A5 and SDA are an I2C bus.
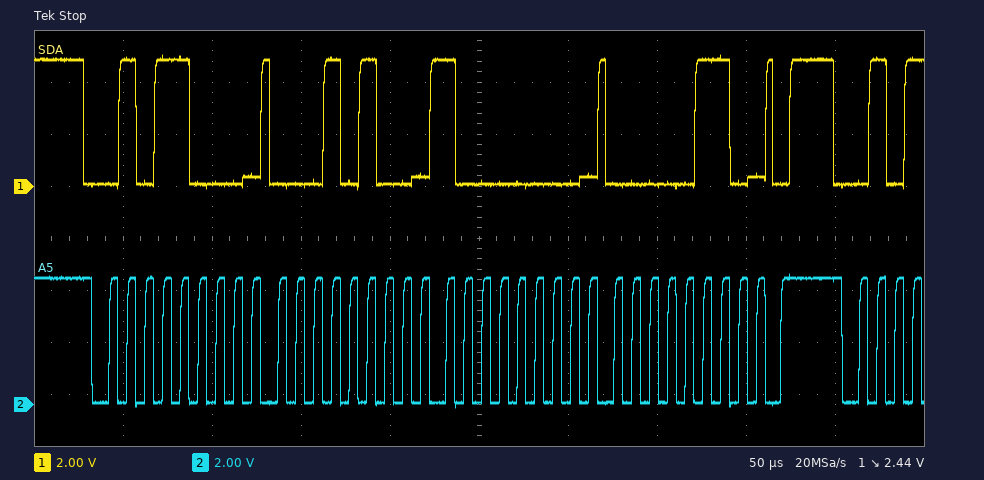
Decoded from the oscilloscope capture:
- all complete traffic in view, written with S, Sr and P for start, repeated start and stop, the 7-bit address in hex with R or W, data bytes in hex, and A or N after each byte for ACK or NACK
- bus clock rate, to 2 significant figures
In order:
S 2CW A 14 A 80 A 06 A P
100 kHz
